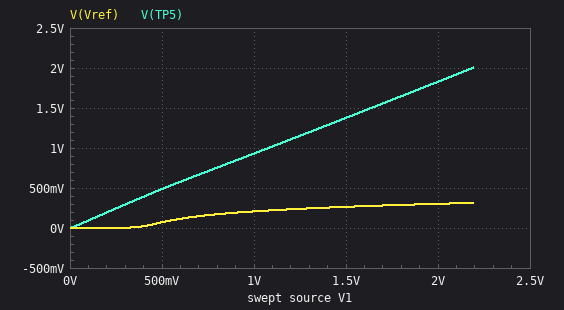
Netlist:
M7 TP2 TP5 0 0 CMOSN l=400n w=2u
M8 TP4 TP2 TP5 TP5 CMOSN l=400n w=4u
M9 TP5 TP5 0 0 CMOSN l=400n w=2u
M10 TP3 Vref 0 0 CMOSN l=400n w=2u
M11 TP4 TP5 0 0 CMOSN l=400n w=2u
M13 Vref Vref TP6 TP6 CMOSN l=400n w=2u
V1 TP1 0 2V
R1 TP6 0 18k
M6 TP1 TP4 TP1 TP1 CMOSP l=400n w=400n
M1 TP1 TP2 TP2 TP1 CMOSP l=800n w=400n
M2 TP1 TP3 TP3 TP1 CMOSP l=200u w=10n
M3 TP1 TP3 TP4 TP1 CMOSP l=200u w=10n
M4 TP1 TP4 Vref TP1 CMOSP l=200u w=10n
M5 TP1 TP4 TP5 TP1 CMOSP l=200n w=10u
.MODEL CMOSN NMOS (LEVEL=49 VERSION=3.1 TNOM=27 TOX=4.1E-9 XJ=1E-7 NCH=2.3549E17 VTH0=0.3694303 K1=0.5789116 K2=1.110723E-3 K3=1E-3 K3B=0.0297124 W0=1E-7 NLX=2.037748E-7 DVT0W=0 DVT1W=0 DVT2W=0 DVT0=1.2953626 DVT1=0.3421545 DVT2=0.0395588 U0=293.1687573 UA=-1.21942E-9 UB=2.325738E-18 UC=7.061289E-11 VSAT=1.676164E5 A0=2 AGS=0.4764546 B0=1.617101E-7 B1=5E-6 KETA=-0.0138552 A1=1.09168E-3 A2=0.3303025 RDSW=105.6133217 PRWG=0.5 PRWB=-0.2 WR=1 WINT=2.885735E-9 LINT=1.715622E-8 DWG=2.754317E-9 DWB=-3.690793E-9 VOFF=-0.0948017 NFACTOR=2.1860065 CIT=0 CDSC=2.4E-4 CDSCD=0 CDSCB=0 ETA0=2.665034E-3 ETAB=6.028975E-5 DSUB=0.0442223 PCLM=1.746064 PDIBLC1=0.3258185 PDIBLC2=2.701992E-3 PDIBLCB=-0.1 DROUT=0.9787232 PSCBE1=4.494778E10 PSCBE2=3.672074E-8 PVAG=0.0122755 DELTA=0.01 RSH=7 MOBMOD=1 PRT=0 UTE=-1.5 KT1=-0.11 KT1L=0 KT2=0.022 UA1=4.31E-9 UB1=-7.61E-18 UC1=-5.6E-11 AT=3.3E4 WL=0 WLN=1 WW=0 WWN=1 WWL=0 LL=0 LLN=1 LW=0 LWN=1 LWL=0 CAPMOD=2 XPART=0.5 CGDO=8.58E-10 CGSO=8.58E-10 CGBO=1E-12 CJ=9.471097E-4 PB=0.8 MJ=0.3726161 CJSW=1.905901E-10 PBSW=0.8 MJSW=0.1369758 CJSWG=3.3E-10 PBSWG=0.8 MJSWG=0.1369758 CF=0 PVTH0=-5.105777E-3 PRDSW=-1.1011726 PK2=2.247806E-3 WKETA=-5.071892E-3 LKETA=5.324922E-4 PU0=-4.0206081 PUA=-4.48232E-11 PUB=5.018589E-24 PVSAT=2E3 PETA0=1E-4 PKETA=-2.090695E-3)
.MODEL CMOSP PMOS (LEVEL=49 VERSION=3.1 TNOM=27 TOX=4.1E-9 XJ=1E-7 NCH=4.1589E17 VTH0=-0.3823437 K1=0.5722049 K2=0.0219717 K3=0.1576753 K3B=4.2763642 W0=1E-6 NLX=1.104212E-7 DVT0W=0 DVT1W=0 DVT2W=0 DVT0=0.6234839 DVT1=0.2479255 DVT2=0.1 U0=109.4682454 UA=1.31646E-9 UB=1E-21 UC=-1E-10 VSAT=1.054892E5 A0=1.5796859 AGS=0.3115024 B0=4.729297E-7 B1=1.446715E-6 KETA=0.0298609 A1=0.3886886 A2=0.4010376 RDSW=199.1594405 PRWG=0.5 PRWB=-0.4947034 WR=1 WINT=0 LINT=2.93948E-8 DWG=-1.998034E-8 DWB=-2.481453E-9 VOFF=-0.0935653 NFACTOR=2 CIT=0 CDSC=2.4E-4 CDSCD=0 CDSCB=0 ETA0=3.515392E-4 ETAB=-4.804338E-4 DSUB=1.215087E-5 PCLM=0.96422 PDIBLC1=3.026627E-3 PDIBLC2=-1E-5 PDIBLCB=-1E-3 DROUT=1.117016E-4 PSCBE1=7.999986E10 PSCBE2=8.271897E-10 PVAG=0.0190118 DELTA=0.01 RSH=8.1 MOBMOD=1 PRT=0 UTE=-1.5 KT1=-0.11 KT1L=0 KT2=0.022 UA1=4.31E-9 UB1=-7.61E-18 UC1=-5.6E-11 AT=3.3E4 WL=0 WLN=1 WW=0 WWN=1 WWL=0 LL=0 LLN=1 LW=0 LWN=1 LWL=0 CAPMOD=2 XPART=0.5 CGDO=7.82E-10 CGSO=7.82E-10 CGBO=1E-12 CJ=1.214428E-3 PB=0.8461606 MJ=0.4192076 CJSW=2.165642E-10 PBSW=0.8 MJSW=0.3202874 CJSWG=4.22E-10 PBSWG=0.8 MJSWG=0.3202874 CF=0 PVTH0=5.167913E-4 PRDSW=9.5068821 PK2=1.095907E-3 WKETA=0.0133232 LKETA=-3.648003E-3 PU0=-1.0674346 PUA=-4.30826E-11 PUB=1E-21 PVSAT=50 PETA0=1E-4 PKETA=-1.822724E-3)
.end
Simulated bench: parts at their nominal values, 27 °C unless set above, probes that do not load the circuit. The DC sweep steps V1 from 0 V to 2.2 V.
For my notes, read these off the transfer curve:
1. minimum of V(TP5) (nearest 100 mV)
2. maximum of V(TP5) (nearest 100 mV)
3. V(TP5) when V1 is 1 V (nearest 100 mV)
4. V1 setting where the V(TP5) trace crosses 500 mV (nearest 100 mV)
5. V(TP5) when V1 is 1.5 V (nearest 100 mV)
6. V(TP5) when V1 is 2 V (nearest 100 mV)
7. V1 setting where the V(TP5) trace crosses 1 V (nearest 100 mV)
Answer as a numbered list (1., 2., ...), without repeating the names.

1. 0 V
2. 2.0 V
3. 900 mV
4. 500 mV
5. 1.4 V
6. 1.8 V
7. 1.1 V
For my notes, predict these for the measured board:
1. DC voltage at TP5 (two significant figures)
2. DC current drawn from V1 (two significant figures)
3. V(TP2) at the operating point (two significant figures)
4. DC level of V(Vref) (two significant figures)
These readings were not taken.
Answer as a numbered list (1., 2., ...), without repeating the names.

1. 1.8 V
2. 710 µA
3. 20 mV
4. 300 mV
